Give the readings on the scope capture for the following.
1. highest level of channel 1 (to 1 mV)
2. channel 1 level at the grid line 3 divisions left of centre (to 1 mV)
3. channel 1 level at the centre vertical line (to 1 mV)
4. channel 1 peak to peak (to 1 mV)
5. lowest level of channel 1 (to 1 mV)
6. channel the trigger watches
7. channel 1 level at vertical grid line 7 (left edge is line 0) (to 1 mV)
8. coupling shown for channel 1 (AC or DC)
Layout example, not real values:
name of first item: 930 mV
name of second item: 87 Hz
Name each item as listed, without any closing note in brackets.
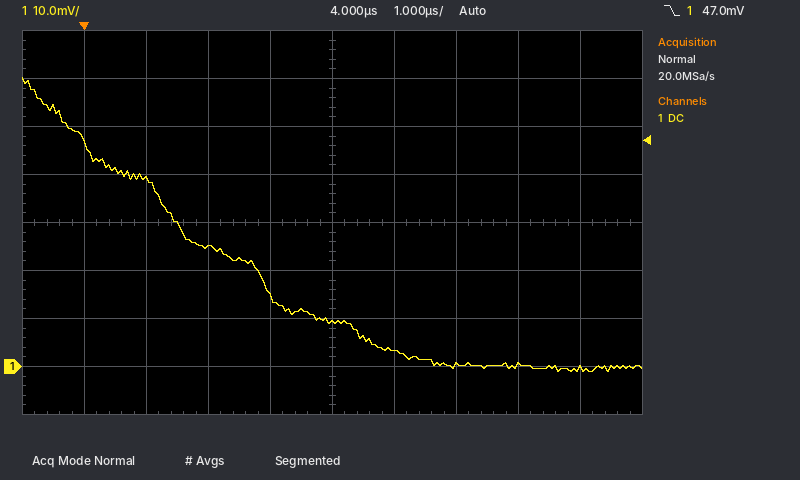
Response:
highest level of channel 1: 60 mV
channel 1 level at the grid line 3 divisions left of centre: 39 mV
channel 1 level at the centre vertical line: 9 mV
channel 1 peak to peak: 61 mV
lowest level of channel 1: -1 mV
channel the trigger watches: channel 1
channel 1 level at vertical grid line 7 (left edge is line 0): 0 mV
coupling shown for channel 1: DC
